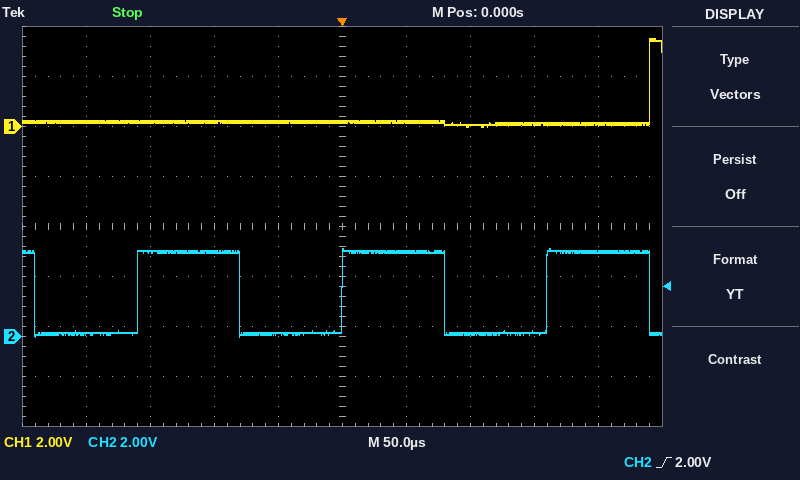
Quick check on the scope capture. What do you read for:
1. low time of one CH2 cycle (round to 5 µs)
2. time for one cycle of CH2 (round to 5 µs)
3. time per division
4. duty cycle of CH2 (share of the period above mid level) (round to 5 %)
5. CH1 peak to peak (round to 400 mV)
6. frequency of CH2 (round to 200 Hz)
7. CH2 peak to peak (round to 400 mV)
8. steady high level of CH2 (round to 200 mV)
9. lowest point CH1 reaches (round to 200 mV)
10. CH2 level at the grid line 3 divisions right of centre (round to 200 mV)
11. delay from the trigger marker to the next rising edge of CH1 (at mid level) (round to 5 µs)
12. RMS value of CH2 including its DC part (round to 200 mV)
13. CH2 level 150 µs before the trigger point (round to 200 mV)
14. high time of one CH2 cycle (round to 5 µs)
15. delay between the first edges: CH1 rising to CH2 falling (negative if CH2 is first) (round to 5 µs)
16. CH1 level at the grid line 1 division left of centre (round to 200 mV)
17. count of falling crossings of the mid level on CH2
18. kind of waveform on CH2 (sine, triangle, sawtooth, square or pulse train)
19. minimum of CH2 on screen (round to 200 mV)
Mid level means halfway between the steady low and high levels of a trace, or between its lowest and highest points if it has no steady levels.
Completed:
80 µs
160 µs
50 µs
50 %
3.6 V
6.2 kHz
3.6 V
3.4 V
0.0 V
200 mV
240 µs
2.4 V
3.4 V
80 µs
-480 µs
200 mV
4
square
0.0 V
